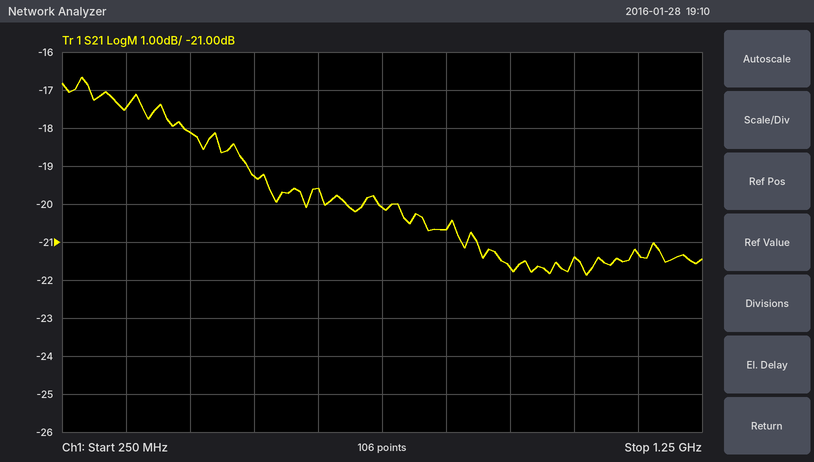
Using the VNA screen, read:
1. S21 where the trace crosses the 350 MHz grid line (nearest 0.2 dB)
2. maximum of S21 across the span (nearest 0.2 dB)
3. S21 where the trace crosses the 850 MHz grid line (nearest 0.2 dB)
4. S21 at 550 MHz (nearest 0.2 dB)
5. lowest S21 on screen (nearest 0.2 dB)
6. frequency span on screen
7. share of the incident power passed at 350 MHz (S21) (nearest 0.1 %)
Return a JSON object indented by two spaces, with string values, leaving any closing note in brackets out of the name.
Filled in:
{
  "S21 where the trace crosses the 350 MHz grid line": "-17.4 dB",
  "maximum of S21 across the span": "-16.6 dB",
  "S21 where the trace crosses the 850 MHz grid line": "-20.6 dB",
  "S21 at 550 MHz": "-19.2 dB",
  "lowest S21 on screen": "-21.8 dB",
  "frequency span on screen": "1 GHz",
  "share of the incident power passed at 350 MHz (S21)": "1.8 %"
}
